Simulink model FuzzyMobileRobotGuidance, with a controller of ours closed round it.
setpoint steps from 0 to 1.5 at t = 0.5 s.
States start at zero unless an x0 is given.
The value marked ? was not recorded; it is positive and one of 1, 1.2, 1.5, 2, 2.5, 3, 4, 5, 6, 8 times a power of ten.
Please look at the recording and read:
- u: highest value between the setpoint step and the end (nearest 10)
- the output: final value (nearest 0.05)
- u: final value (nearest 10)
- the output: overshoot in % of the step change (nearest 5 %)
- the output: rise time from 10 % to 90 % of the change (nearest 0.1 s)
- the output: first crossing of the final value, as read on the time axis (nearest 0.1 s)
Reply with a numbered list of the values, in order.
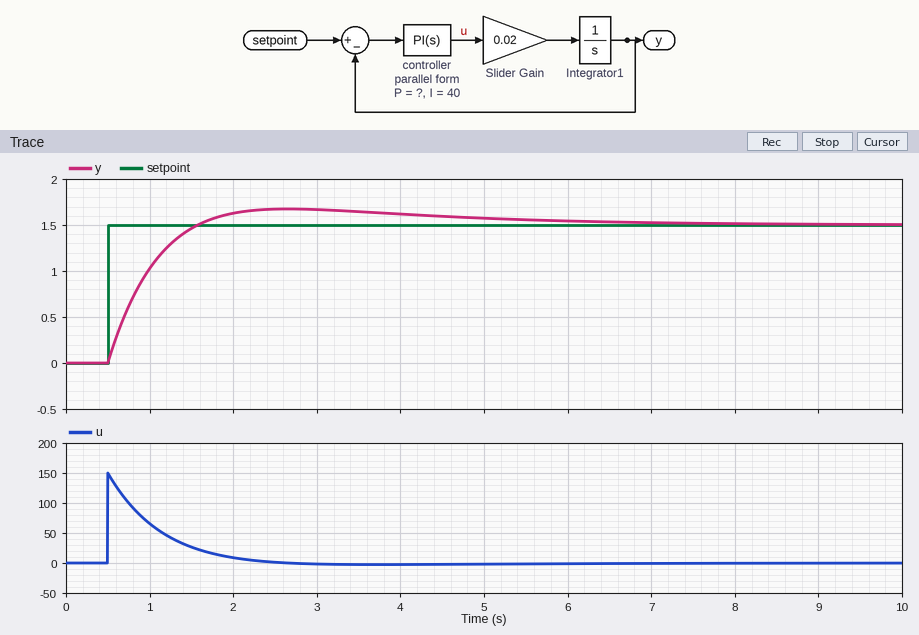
1. 150
2. 1.50
3. 0
4. 10 %
5. 0.8 s
6. 1.6 s
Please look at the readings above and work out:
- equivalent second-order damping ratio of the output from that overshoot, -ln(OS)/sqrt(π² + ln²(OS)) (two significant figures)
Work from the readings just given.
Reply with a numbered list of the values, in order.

1. 0.59
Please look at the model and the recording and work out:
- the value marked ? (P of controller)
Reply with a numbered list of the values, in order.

1. 100
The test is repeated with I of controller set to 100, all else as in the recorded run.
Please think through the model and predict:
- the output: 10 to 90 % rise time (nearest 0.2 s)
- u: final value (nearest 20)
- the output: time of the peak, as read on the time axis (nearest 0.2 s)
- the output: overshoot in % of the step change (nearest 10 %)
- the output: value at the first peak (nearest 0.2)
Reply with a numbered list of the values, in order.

1. 0.6 s
2. 0
3. 2.0 s
4. 20 %
5. 1.8
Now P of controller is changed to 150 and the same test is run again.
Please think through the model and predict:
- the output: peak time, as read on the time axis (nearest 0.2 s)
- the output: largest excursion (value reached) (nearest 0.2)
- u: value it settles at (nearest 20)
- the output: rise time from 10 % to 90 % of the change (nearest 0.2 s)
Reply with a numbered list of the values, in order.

1. 2.4 s
2. 1.6
3. 0
4. 0.6 s
